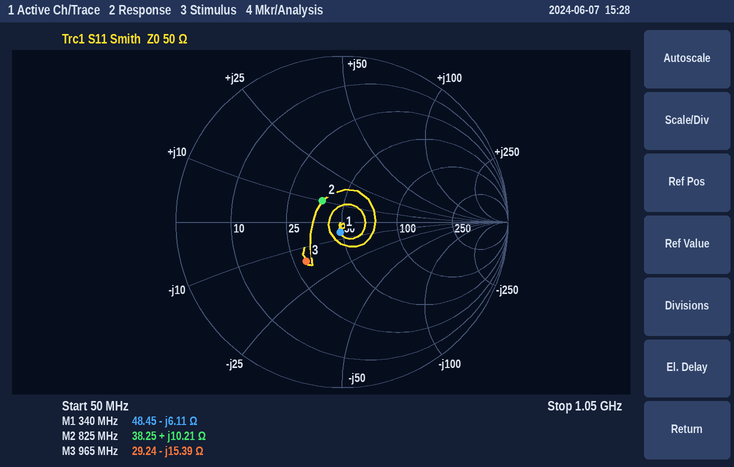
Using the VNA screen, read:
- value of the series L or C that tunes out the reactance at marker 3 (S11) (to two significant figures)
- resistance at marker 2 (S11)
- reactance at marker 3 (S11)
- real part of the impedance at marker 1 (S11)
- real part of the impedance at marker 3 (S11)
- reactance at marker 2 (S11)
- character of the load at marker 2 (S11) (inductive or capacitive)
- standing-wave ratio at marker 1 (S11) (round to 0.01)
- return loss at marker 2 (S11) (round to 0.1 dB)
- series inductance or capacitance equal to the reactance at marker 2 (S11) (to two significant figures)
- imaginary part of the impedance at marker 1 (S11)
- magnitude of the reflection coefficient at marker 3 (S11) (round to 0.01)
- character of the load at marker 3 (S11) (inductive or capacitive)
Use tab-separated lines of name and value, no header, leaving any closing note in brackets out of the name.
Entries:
value of the series L or C that tunes out the reactance at marker 3 (S11)	2.5 nH
resistance at marker 2	38.25 Ω
reactance at marker 3	-15.39 Ω
real part of the impedance at marker 1	48.45 Ω
real part of the impedance at marker 3	29.24 Ω
reactance at marker 2	+10.21 Ω
character of the load at marker 2 (S11)	inductive
standing-wave ratio at marker 1 (S11)	1.14
return loss at marker 2 (S11)	15.1 dB
series inductance or capacitance equal to the reactance at marker 2 (S11)	2.0 nH
imaginary part of the impedance at marker 1	-6.11 Ω
magnitude of the reflection coefficient at marker 3 (S11)	0.32
character of the load at marker 3 (S11)	capacitive
